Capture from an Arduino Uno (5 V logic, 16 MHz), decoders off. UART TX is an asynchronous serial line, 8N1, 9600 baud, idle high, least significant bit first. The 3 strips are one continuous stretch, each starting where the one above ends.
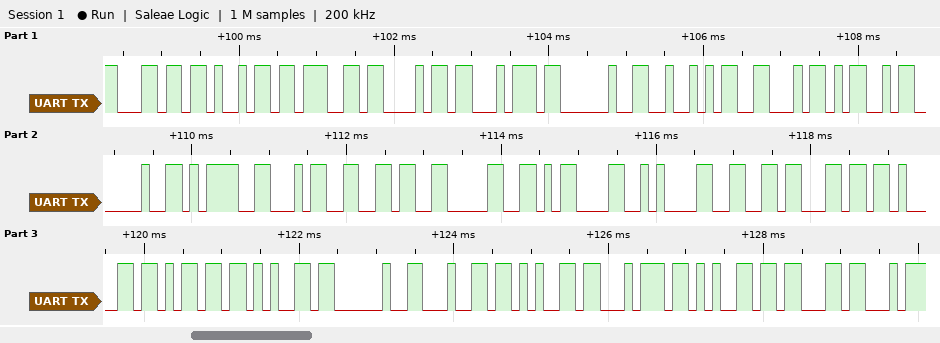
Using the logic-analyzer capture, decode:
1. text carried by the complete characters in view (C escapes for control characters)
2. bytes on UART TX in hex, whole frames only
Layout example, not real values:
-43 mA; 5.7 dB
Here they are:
"light RFM =460\r\nflame detec"; 6C 69 67 68 74 20 52 46 4D 20 3D 34 36 30 0D 0A 66 6C 61 6D 65 20 64 65 74 65 63
